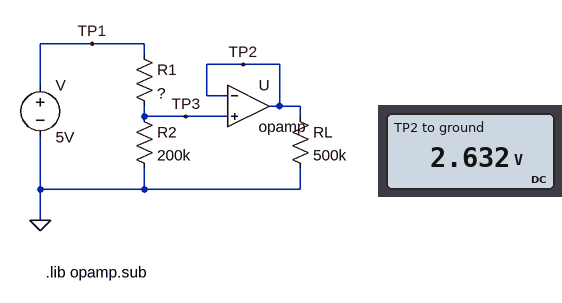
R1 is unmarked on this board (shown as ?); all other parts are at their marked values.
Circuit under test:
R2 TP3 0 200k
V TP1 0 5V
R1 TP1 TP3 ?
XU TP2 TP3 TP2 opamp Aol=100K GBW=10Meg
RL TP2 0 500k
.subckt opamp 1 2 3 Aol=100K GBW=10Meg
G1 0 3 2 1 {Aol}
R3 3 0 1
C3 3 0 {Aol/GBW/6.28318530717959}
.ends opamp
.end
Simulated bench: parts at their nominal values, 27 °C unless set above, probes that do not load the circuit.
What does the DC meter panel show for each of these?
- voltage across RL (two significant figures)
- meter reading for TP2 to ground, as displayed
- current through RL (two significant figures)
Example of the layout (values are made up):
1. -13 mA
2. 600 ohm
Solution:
1. 2.6 V
2. 2.632 V
3. 5.3 µA
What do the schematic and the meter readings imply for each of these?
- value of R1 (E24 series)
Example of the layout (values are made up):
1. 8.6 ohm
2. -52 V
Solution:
1. 180 kΩ
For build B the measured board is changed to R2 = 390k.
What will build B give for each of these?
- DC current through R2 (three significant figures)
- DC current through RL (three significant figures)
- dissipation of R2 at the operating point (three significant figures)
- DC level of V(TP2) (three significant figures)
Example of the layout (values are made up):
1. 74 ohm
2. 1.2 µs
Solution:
1. 8.77 µA
2. 6.84 µA
3. 30.0 µW
4. 3.42 V
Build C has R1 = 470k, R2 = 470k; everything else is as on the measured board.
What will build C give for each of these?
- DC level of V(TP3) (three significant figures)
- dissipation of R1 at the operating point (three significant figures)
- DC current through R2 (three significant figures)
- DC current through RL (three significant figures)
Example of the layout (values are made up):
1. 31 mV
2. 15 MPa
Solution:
1. 2.50 V
2. 13.3 µW
3. 5.32 µA
4. 5.00 µA
